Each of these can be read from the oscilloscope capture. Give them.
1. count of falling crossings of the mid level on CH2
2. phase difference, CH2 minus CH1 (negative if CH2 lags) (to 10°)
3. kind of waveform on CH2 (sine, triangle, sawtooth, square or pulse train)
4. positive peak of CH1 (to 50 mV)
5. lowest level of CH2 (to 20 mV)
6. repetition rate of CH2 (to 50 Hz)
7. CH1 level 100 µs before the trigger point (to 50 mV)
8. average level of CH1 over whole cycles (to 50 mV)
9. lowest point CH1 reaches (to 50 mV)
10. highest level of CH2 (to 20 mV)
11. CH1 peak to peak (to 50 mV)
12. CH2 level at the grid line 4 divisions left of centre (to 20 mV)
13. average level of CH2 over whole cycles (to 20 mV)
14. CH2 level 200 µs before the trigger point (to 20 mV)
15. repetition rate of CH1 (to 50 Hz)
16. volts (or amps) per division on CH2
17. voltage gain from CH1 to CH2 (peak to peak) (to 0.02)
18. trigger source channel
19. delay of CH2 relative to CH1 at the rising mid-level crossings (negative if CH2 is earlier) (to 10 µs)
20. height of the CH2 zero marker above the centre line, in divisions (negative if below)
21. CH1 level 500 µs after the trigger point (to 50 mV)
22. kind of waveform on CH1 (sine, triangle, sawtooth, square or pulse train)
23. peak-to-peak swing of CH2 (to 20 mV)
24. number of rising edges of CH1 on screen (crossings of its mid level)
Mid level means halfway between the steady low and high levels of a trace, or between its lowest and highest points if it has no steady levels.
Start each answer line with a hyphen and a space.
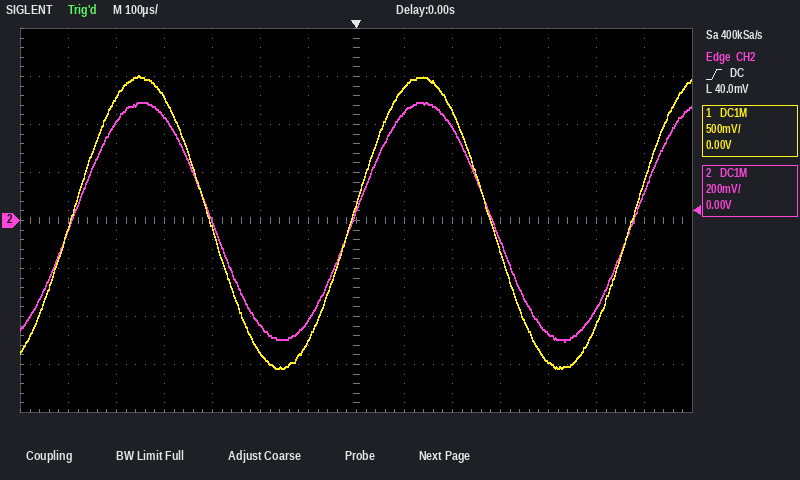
- 2
- 0°
- sine
- 1.50 V
- -500 mV
- 1.70 kHz
- -1.25 V
- 0 mV
- -1.55 V
- 500 mV
- 3.05 V
- 440 mV
- 0 mV
- -440 mV
- 1.70 kHz
- 200 mV
- 0.32
- CH2
- 0 µs
- 0.0 div
- -1.10 V
- sine
- 1.00 V
- 3
